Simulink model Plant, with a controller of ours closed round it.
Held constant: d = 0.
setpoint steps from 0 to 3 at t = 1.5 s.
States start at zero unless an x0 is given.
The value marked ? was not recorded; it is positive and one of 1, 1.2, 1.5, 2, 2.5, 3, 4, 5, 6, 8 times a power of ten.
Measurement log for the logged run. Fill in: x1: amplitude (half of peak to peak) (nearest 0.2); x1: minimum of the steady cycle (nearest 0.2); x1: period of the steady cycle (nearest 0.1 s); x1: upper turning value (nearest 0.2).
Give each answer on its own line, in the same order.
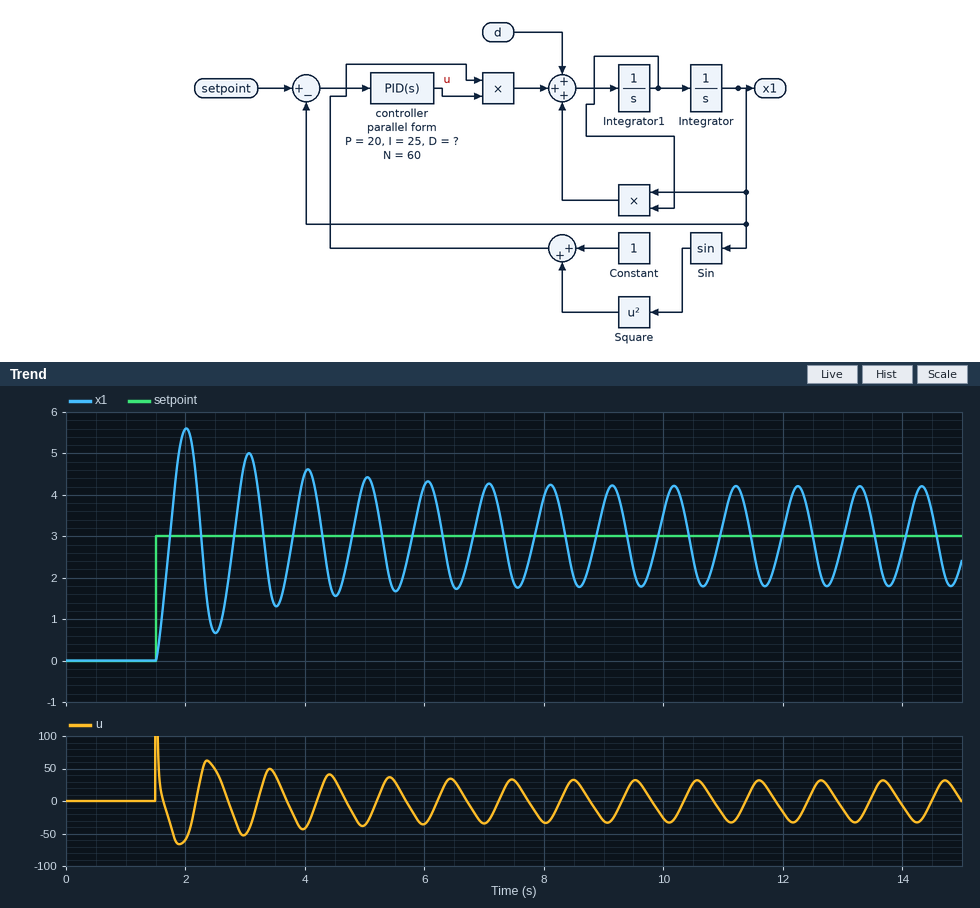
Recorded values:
1.2
1.8
1.0 s
4.2
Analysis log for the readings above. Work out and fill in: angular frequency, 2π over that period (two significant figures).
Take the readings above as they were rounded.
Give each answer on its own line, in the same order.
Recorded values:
6.3 rad/s
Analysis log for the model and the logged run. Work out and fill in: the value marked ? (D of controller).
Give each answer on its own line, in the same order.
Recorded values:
3
